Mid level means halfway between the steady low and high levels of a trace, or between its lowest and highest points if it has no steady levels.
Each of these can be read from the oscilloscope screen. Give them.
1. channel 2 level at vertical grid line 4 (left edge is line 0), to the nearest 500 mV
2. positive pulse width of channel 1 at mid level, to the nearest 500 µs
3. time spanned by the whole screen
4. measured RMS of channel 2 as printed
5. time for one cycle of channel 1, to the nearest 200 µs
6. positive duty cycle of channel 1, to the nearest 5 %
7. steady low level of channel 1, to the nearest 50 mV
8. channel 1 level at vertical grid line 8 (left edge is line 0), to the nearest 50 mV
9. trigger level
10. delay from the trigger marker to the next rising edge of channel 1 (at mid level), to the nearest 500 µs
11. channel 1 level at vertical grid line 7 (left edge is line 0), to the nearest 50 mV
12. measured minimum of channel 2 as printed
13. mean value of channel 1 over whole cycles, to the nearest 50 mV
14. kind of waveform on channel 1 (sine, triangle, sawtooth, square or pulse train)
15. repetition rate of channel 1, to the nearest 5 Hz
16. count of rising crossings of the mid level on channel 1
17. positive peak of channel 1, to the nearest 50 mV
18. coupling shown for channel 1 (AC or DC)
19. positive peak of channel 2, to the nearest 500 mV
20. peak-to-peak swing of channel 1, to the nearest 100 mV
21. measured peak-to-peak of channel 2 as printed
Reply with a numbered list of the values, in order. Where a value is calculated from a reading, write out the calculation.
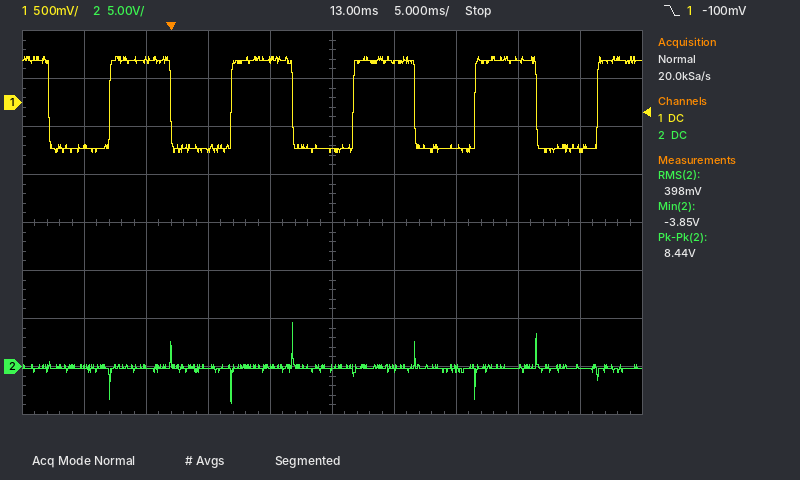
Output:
1. 0.0 V
2. 5.0 ms
3. 50 ms
4. 398 mV
5. 9.8 ms
6. 5.0 ms / 9.8 ms ≈ 51.0 %, so 50 % to the nearest 5 %
7. -500 mV
8. 450 mV
9. -100 mV
10. 5.0 ms
11. -450 mV
12. -3.85 V
13. -500 mV + 0.5 × (500 mV − (-500 mV)) ≈ 0 mV
14. square
15. 1 / 9.8 ms ≈ 102 Hz, so 100 Hz to the nearest 5 Hz
16. 5
17. 500 mV
18. DC
19. 4.5 V
20. 1.00 V
21. 8.44 V
